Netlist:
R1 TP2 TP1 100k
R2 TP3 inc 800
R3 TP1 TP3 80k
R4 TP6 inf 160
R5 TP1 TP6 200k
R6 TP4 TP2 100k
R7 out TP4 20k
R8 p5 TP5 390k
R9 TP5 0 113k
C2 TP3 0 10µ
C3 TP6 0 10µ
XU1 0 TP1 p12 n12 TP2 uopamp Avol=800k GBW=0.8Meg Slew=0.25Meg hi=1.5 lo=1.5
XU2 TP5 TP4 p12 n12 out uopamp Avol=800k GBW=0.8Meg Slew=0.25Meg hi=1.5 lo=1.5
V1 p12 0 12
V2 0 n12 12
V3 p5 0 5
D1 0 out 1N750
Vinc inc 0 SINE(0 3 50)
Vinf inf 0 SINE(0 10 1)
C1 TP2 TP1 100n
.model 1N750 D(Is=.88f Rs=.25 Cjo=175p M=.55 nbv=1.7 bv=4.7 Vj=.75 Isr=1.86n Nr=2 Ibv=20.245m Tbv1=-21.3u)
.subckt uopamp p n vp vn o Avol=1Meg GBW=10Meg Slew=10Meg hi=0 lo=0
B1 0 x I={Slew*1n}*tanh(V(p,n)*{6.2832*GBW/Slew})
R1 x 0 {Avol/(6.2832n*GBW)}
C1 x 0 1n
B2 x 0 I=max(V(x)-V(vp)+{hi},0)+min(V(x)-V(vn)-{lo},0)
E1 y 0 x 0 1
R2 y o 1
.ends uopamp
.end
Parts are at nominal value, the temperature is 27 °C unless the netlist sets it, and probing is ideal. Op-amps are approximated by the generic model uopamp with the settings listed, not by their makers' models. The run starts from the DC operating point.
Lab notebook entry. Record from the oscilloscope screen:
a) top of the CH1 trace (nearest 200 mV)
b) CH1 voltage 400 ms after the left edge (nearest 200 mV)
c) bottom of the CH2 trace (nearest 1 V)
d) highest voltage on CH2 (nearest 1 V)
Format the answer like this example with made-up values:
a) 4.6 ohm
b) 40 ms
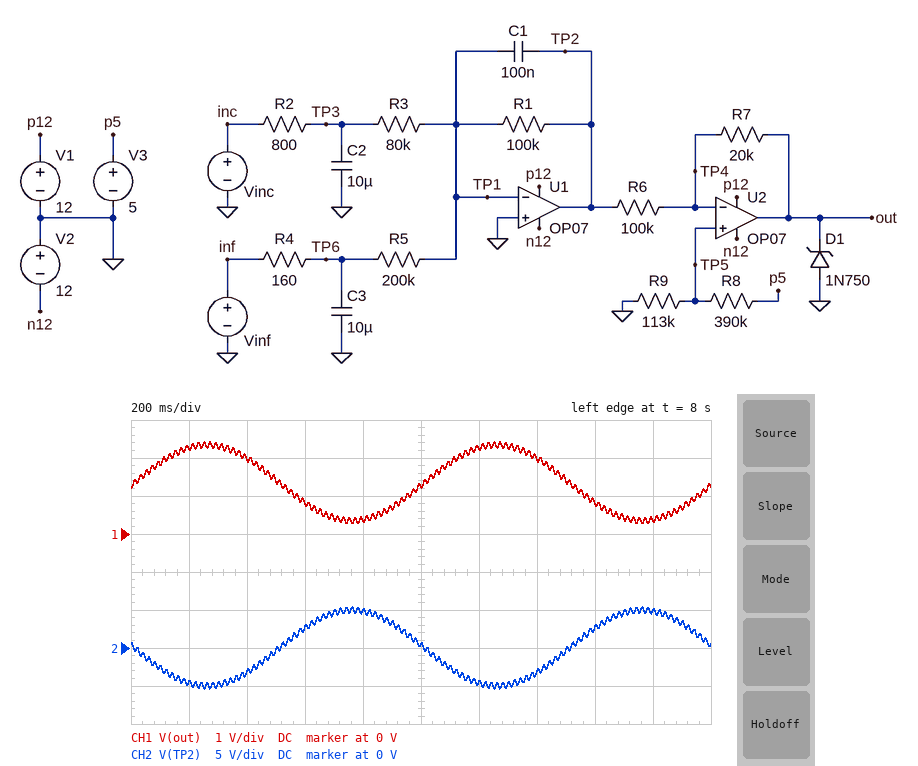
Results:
a) 2.4 V
b) 2.0 V
c) -5 V
d) 5 V
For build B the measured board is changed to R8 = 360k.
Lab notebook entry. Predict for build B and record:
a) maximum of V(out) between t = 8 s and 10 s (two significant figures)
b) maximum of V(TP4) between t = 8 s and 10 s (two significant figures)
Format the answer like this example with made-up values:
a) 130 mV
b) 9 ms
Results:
a) 2.5 V
b) 1.2 V
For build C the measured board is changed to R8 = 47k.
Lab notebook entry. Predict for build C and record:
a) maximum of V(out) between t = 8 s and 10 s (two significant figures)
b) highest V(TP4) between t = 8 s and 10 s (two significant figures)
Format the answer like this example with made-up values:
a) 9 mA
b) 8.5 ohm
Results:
a) 5.3 V
b) 3.5 V
